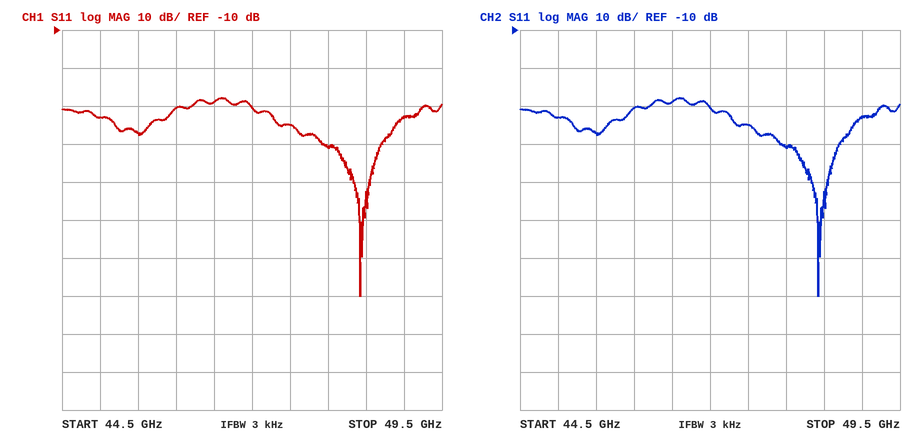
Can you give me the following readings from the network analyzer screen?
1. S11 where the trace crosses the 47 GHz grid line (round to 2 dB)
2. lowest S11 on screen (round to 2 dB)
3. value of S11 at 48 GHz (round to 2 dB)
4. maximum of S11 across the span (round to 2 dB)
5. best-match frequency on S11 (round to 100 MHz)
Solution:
-30 dB
-80 dB
-40 dB
-28 dB
48.4 GHz
